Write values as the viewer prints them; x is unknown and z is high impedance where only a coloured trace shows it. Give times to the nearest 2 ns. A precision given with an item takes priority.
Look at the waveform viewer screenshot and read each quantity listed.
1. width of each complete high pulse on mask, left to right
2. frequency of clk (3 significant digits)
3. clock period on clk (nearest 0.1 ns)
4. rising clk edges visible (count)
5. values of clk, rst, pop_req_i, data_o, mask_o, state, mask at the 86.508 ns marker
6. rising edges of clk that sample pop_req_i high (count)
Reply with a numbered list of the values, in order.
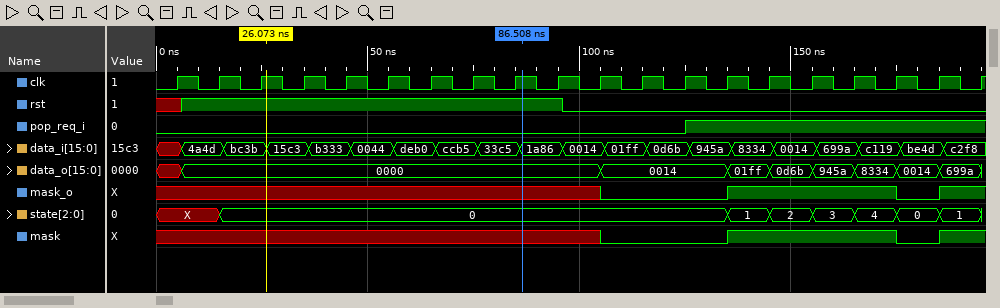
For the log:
1. 40 ns
2. 100 MHz
3. 10 ns
4. 20
5. clk=1, rst=1, pop_req_i=0, data_o=0000, mask_o=x, state=0, mask=x
6. 7
